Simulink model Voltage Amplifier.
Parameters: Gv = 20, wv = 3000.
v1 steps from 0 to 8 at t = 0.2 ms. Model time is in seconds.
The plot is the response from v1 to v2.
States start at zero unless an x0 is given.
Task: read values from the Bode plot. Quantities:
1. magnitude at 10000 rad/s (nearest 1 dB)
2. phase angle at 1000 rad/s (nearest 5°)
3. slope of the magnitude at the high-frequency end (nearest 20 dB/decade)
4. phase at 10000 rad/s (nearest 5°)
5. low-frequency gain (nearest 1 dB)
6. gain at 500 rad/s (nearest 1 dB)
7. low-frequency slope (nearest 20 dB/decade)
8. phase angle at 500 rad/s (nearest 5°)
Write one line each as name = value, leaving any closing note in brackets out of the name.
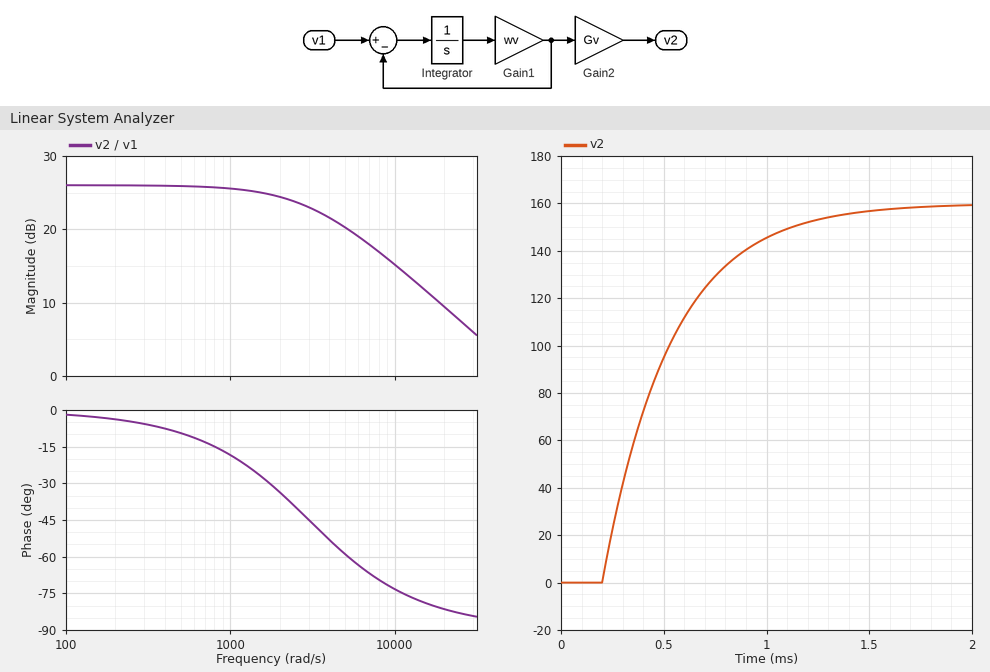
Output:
magnitude at 10000 rad/s = 15 dB
phase angle at 1000 rad/s = -20°
slope of the magnitude at the high-frequency end = -20 dB/decade
phase at 10000 rad/s = -75°
low-frequency gain = 26 dB
gain at 500 rad/s = 26 dB
low-frequency slope = 0 dB/decade
phase angle at 500 rad/s = -10°
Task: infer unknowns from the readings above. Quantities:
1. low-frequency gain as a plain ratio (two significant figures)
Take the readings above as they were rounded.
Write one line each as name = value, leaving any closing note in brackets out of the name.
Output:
low-frequency gain as a plain ratio = 20
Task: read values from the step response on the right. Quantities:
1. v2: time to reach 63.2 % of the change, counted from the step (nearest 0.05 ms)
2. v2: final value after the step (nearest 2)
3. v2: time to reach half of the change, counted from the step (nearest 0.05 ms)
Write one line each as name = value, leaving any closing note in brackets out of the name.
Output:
v2: time to reach 63.2 % of the change, counted from the step = 0.35 ms
v2: final value after the step = 160
v2: time to reach half of the change, counted from the step = 0.25 ms
